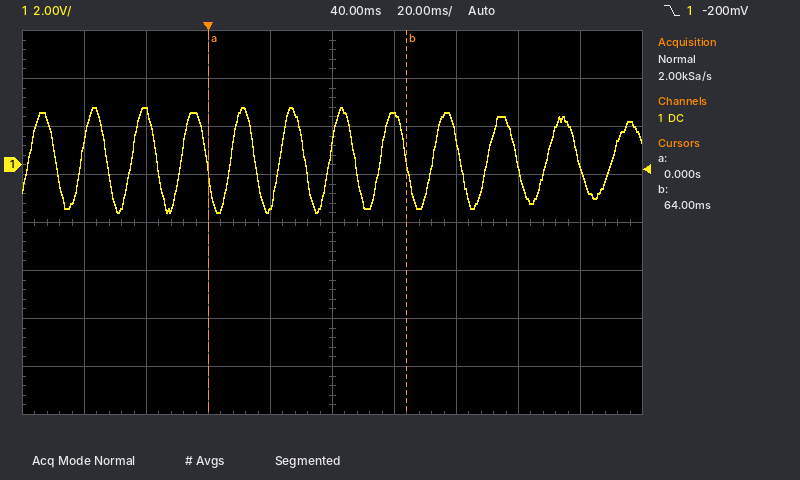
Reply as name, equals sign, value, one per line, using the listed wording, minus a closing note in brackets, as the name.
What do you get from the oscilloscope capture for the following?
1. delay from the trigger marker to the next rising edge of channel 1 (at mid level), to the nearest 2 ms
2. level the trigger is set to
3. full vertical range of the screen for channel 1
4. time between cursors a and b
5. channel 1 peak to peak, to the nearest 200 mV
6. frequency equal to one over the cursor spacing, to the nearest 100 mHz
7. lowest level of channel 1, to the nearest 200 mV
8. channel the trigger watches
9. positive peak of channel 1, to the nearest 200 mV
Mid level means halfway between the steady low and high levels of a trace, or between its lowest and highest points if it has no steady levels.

delay from the trigger marker to the next rising edge of channel 1 (at mid level), to the nearest 2 ms = 8 ms
level the trigger is set to = -200 mV
full vertical range of the screen for channel 1 = 16 V
time between cursors a and b = 64 ms
channel 1 peak to peak, to the nearest 200 mV = 4.4 V
frequency equal to one over the cursor spacing, to the nearest 100 mHz = 15.6 Hz
lowest level of channel 1, to the nearest 200 mV = -2.0 V
channel the trigger watches = channel 1
positive peak of channel 1, to the nearest 200 mV = 2.4 V
